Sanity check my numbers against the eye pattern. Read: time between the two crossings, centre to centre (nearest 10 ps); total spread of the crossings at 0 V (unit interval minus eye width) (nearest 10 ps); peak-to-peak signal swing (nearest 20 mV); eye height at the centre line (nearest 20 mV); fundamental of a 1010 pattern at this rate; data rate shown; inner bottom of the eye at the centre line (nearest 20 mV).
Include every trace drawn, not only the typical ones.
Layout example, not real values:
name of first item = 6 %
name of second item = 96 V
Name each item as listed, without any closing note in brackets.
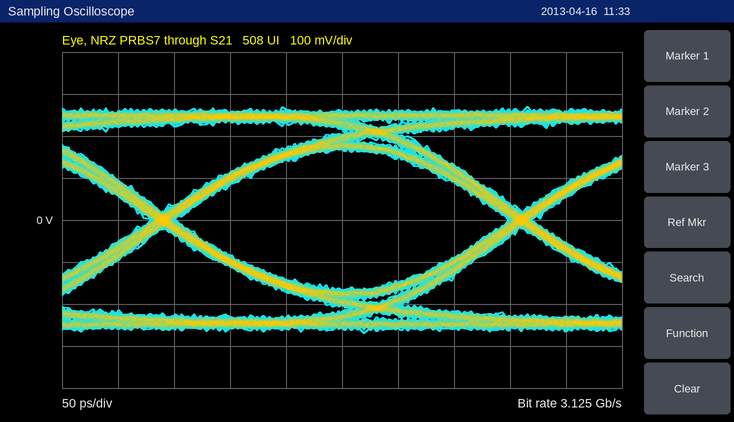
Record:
time between the two crossings, centre to centre = 320 ps
total spread of the crossings at 0 V (unit interval minus eye width) = 20 ps
peak-to-peak signal swing = 540 mV
eye height at the centre line = 340 mV
fundamental of a 1010 pattern at this rate = 1.5625 GHz
data rate shown = 3.125 Gb/s
inner bottom of the eye at the centre line = -160 mV
